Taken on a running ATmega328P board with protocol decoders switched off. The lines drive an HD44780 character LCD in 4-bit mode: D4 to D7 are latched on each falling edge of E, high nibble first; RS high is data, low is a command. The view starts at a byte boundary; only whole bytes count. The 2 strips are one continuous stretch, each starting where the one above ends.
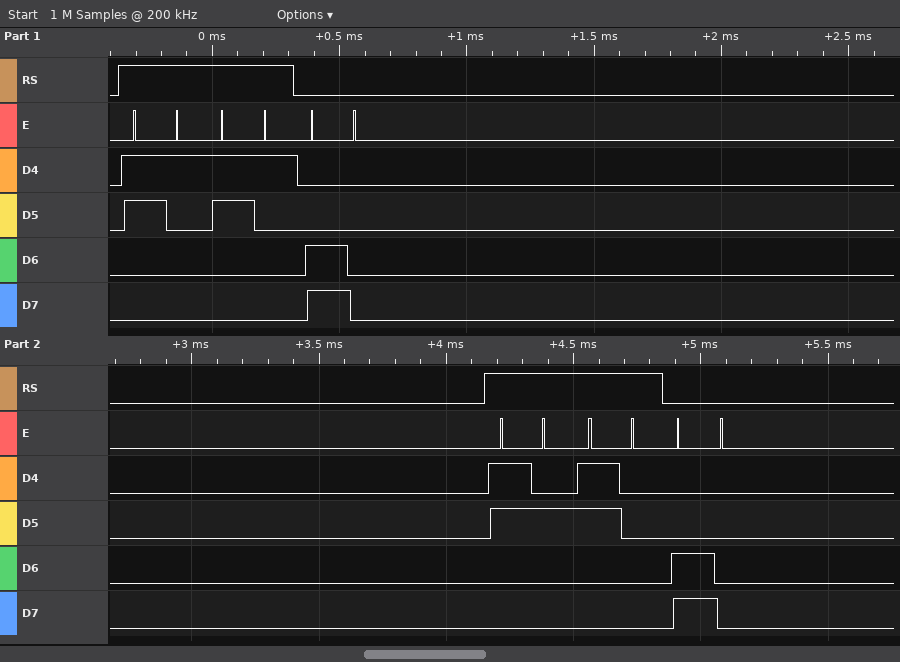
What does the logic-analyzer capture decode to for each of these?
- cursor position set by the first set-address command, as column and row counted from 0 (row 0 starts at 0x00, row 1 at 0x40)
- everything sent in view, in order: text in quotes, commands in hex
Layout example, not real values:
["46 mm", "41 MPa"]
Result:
["column 0, row 1", "\"11\" 0xC0 \"20\" 0xC0"]
